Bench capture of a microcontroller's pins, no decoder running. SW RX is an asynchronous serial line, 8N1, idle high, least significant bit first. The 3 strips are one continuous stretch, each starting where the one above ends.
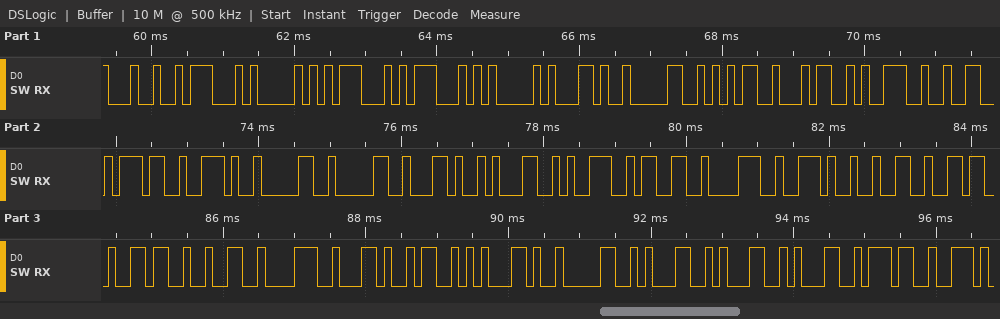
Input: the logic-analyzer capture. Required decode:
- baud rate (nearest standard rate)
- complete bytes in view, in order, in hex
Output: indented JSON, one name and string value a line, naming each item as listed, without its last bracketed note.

{
  "baud rate": "9600 baud",
  "complete bytes in view, in order, in hex": "24 47 50 47 47 41 2C 30 35 34 39 32 37 2E 30 30 2C 31 39 33 38 2E 32 36 36 32 38 2C 53 2C 30 31 31 31 37"
}
